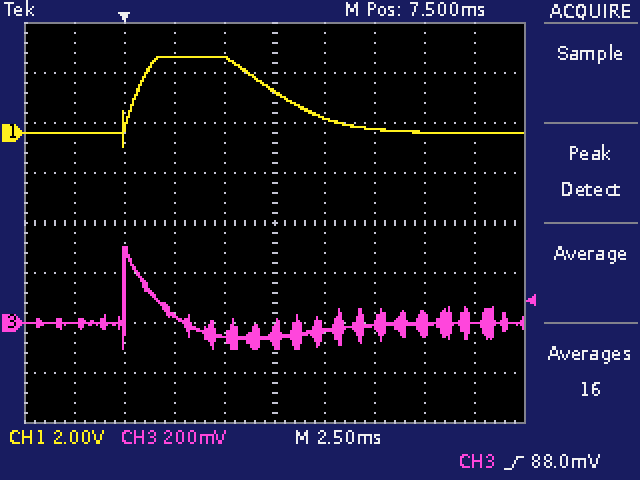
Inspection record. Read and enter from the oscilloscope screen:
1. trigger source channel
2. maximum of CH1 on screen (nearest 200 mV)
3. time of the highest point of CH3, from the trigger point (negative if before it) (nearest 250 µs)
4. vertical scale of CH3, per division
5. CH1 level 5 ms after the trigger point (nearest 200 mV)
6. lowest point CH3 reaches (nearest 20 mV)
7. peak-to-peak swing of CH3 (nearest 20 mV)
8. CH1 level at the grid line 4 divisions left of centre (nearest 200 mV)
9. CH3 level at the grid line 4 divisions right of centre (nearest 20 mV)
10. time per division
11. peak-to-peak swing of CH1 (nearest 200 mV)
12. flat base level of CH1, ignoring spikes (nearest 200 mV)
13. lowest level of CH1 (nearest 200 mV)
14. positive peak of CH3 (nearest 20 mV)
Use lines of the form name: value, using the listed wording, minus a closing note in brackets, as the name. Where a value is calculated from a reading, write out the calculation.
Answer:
trigger source channel: CH3
maximum of CH1 on screen: 3.0 V
time of the highest point of CH3, from the trigger point (negative if before it): 0.00 ms
vertical scale of CH3, per division: 200 mV
CH1 level 5 ms after the trigger point: 3.0 V
lowest point CH3 reaches: -100 mV
peak-to-peak swing of CH3: 300 mV − (-100 mV) = 400 mV
CH1 level at the grid line 4 divisions left of centre: 0.0 V
CH3 level at the grid line 4 divisions right of centre: 0 mV
time per division: 2.5 ms
peak-to-peak swing of CH1: 3.0 V − (-600 mV) = 3.6 V
flat base level of CH1, ignoring spikes: 0.0 V
lowest level of CH1: -600 mV
positive peak of CH3: 300 mV
